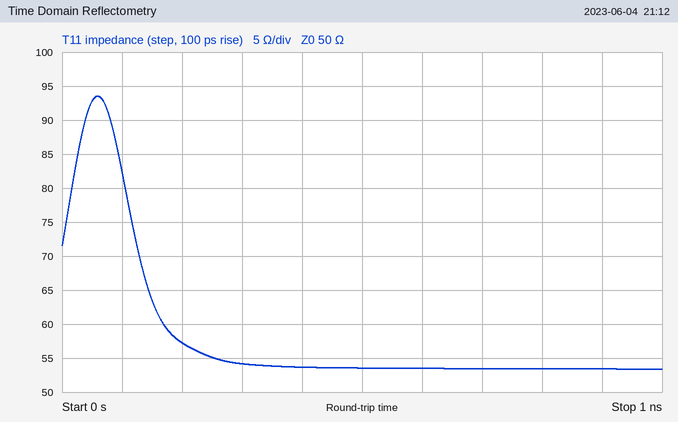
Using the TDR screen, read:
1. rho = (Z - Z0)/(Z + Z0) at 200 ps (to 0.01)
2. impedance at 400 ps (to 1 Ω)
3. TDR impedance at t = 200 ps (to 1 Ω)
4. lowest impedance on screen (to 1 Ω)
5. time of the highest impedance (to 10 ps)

+0.07
54 Ω
57 Ω
53 Ω
60 ps
